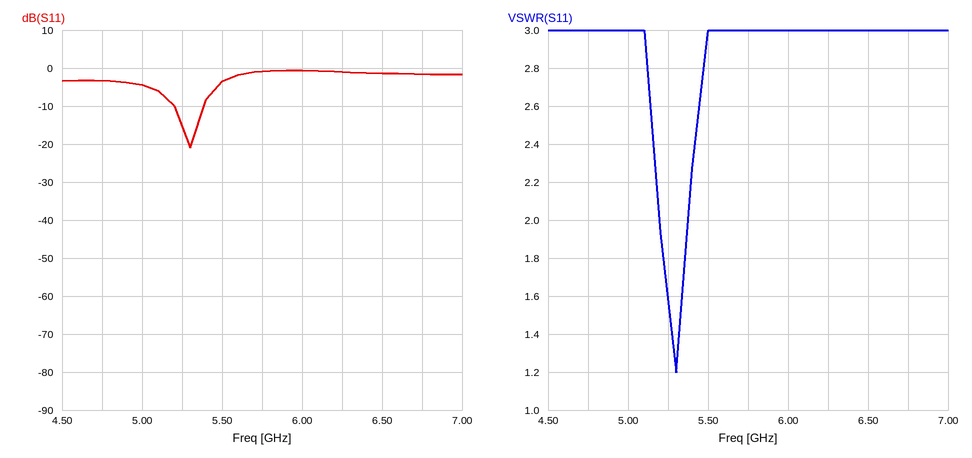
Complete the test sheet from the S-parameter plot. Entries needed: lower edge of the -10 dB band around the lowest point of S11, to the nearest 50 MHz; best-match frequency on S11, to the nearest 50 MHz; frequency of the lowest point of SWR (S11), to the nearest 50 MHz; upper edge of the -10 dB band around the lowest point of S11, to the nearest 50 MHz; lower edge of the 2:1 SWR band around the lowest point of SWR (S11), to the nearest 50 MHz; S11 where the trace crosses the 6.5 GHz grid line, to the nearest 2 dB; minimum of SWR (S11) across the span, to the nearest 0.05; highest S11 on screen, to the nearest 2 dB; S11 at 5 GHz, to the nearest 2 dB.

5.20 GHz
5.30 GHz
5.30 GHz
5.40 GHz
5.20 GHz
-2 dB
1.20
0 dB
-4 dB
